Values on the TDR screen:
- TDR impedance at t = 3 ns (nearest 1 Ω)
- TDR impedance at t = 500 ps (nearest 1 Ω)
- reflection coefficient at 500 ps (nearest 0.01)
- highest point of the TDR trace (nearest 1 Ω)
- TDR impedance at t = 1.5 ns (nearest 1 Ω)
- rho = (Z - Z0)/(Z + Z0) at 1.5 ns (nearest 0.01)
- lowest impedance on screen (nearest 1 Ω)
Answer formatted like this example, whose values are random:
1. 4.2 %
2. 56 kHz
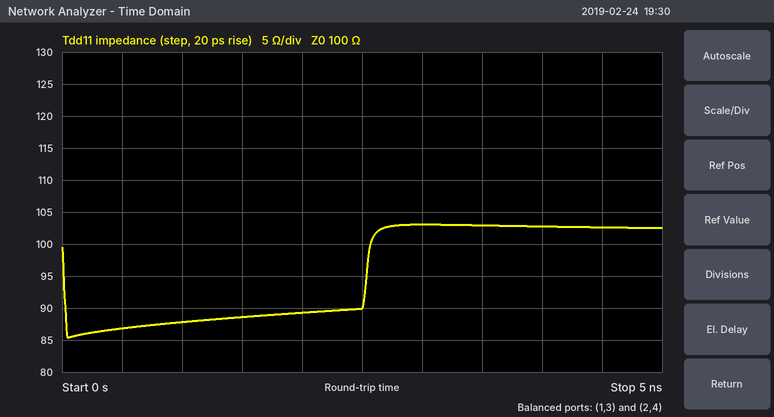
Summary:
1. 103 Ω
2. 87 Ω
3. -0.07
4. 103 Ω
5. 89 Ω
6. -0.06
7. 85 Ω
